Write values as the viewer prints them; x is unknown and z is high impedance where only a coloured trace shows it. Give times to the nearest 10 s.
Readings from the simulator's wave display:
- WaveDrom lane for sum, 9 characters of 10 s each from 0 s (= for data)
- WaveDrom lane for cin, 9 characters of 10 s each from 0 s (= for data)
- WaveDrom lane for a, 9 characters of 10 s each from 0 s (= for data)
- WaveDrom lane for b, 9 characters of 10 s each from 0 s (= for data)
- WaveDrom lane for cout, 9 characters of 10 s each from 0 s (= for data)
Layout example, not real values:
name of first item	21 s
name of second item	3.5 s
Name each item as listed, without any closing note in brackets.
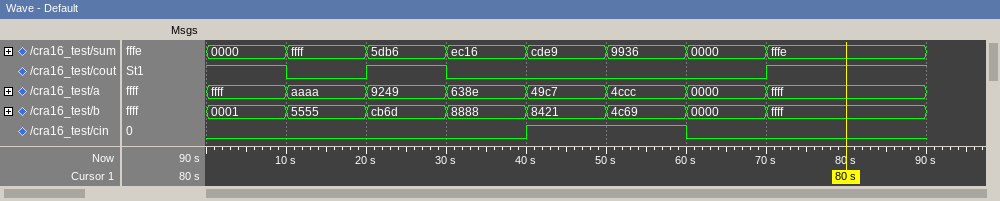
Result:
WaveDrom lane for sum, 9 characters of 10 s each from 0 s	{name: 'sum', wave: '========.', data: '0000 ffff 5db6 ec16 cde9 9936 0000 fffe'}
WaveDrom lane for cin, 9 characters of 10 s each from 0 s	{name: 'cin', wave: '0...1.0..'}
WaveDrom lane for a, 9 characters of 10 s each from 0 s	{name: 'a', wave: '========.', data: 'ffff aaaa 9249 638e 49c7 4ccc 0000 ffff'}
WaveDrom lane for b, 9 characters of 10 s each from 0 s	{name: 'b', wave: '========.', data: '0001 5555 cb6d 8888 8421 4c69 0000 ffff'}
WaveDrom lane for cout, 9 characters of 10 s each from 0 s	{name: 'cout', wave: '1010...1.'}
